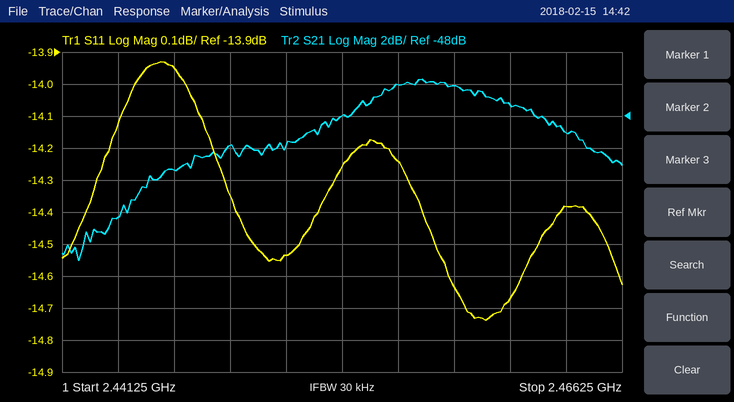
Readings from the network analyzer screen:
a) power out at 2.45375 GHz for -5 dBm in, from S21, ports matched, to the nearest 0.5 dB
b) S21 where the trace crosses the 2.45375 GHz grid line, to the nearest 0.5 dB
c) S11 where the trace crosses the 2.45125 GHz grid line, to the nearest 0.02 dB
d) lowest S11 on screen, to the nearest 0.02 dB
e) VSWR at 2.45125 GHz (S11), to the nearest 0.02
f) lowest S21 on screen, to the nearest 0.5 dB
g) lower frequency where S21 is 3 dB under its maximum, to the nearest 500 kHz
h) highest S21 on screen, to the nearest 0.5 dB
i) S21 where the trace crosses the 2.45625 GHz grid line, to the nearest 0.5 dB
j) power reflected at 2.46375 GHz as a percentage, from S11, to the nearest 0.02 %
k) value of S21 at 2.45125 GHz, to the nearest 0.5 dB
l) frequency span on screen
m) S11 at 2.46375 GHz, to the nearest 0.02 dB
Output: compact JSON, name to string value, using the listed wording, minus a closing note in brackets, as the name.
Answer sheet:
{"power out at 2.45375 GHz for -5 dBm in, from S21, ports matched, to the nearest 0.5 dB": "-53.0 dBm", "S21 where the trace crosses the 2.45375 GHz grid line, to the nearest 0.5 dB": "-48.0 dB", "S11 where the trace crosses the 2.45125 GHz grid line, to the nearest 0.02 dB": "-14.54 dB", "lowest S11 on screen, to the nearest 0.02 dB": "-14.74 dB", "VSWR at 2.45125 GHz (S11), to the nearest 0.02": "1.46", "lowest S21 on screen, to the nearest 0.5 dB": "-57.0 dB", "lower frequency where S21 is 3 dB under its maximum, to the nearest 500 kHz": "2.4530 GHz", "highest S21 on screen, to the nearest 0.5 dB": "-45.5 dB", "S21 where the trace crosses the 2.45625 GHz grid line, to the nearest 0.5 dB": "-46.0 dB", "power reflected at 2.46375 GHz as a percentage, from S11, to the nearest 0.02 %": "3.64 %", "value of S21 at 2.45125 GHz, to the nearest 0.5 dB": "-50.0 dB", "frequency span on screen": "25 MHz", "S11 at 2.46375 GHz, to the nearest 0.02 dB": "-14.38 dB"}
